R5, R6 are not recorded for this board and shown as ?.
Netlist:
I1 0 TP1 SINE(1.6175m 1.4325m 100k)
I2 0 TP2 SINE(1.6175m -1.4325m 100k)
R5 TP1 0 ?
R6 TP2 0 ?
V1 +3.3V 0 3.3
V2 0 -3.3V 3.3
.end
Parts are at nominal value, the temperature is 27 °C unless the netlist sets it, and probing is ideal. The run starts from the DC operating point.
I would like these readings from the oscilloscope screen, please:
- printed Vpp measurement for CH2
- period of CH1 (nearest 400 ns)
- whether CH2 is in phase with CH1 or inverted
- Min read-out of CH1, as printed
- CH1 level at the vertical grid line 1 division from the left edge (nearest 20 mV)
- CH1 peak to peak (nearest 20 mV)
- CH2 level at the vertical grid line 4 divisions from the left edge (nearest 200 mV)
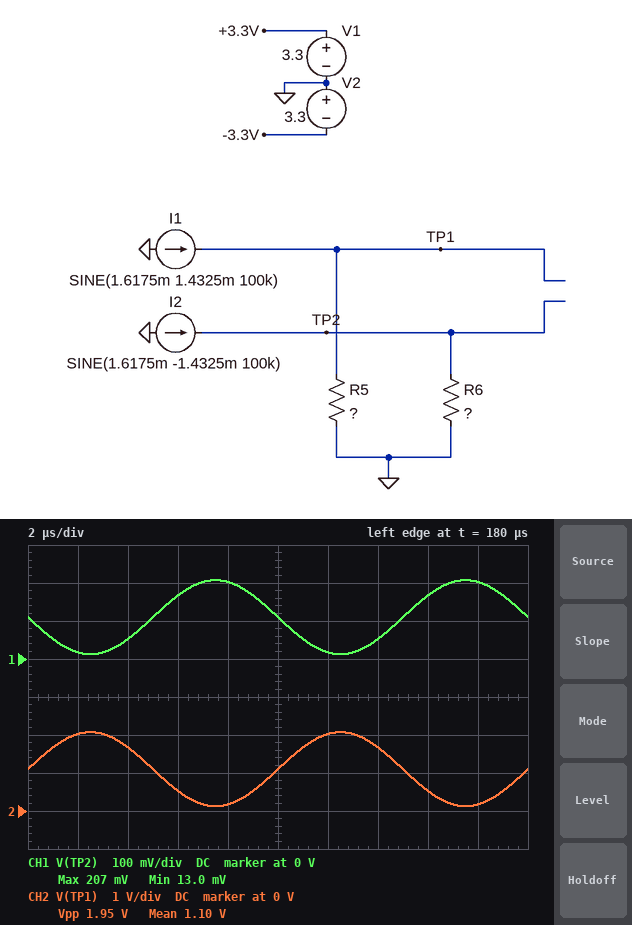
1.95 V
10.0 µs
inverted
13.0 mV
20 mV
200 mV
200 mV
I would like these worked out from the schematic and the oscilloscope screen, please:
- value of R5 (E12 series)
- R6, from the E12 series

680 Ω
68 Ω
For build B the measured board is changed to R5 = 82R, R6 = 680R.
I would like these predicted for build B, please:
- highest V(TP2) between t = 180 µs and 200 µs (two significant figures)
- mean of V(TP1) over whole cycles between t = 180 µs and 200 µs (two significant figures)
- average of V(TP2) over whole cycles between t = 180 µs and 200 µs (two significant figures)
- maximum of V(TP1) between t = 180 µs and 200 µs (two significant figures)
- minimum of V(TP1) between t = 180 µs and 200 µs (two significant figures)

2.1 V
130 mV
1.1 V
250 mV
15 mV
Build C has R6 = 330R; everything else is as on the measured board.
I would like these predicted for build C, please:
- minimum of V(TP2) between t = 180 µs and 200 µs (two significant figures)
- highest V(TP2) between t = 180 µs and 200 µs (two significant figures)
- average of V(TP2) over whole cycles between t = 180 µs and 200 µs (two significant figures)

61 mV
1.0 V
530 mV
